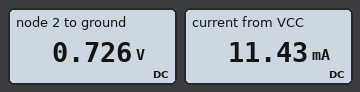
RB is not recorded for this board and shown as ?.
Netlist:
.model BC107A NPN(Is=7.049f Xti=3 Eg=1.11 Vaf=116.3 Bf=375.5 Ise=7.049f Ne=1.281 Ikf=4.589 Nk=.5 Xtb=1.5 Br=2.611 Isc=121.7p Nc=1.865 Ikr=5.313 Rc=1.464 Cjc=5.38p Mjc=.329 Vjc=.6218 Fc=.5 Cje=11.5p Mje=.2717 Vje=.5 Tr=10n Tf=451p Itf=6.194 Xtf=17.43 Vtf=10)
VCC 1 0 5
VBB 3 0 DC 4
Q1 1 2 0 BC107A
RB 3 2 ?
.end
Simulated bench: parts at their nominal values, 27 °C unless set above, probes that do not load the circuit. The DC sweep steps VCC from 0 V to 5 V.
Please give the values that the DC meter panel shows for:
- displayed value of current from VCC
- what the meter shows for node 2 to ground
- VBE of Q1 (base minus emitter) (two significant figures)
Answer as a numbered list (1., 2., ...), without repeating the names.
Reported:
1. 11.43 mA
2. 0.726 V
3. 730 mV
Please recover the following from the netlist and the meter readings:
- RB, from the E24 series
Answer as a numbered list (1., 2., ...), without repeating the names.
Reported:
1. 62 kΩ
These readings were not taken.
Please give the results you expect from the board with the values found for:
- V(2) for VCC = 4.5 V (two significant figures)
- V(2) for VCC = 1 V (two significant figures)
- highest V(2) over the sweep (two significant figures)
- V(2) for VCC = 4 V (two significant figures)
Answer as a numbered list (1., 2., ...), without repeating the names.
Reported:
1. 730 mV
2. 730 mV
3. 730 mV
4. 730 mV
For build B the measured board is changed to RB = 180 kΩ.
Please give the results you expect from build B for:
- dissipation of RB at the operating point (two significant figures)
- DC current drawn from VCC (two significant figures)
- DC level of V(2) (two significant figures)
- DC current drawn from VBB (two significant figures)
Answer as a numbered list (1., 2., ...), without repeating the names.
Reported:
1. 61 µW
2. 3.5 mA
3. 700 mV
4. 18 µA
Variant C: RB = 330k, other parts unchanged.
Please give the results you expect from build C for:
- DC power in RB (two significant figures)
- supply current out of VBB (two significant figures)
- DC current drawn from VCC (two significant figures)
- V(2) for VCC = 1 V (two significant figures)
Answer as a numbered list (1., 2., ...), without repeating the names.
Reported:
1. 33 µW
2. 10 µA
3. 1.8 mA
4. 680 mV
